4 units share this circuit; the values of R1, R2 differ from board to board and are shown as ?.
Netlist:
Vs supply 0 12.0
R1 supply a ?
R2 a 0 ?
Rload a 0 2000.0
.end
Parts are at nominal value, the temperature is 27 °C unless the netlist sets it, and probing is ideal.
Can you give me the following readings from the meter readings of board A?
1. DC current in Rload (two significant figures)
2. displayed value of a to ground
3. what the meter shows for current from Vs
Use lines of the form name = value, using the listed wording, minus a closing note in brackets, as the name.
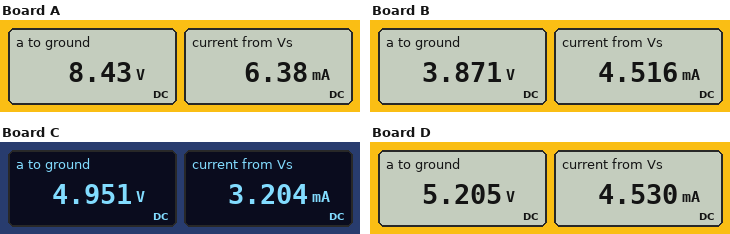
DC current in Rload = 4.2 mA
displayed value of a to ground = 8.43 V
what the meter shows for current from Vs = 6.38 mA
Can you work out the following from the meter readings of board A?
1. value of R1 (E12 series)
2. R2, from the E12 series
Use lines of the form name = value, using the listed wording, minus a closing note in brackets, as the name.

value of R1 = 560 Ω
R2, from the E12 series = 3.9 kΩ
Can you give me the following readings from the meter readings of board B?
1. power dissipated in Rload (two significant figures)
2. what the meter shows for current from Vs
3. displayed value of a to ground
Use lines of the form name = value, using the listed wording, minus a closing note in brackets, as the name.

power dissipated in Rload = 7.5 mW
what the meter shows for current from Vs = 4.516 mA
displayed value of a to ground = 3.871 V
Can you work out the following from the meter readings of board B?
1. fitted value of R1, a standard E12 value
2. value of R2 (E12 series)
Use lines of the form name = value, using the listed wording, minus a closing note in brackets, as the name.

fitted value of R1, a standard E12 value = 1.8 kΩ
value of R2 = 1.5 kΩ
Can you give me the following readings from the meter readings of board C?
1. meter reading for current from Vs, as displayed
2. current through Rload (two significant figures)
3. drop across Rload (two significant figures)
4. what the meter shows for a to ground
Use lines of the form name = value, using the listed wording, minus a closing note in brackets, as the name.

meter reading for current from Vs, as displayed = 3.204 mA
current through Rload = 2.5 mA
drop across Rload = 5.0 V
what the meter shows for a to ground = 4.951 V
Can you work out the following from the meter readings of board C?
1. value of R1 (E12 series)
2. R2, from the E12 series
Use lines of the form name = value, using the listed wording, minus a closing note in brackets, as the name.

value of R1 = 2.2 kΩ
R2, from the E12 series = 6.8 kΩ
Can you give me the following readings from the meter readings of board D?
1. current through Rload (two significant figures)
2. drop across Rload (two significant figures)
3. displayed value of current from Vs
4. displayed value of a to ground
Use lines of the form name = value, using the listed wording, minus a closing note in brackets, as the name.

current through Rload = 2.6 mA
drop across Rload = 5.2 V
displayed value of current from Vs = 4.530 mA
displayed value of a to ground = 5.205 V
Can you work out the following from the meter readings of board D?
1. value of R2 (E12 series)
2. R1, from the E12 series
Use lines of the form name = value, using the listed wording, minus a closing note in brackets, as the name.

value of R2 = 2.7 kΩ
R1, from the E12 series = 1.5 kΩ
